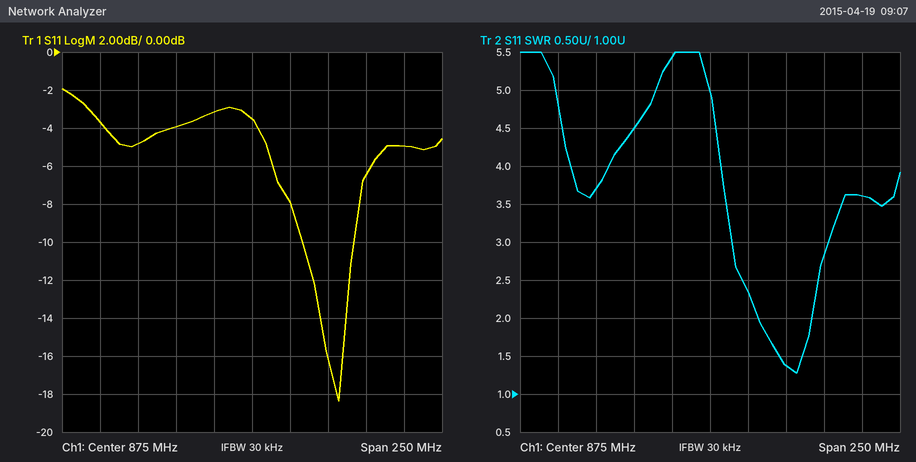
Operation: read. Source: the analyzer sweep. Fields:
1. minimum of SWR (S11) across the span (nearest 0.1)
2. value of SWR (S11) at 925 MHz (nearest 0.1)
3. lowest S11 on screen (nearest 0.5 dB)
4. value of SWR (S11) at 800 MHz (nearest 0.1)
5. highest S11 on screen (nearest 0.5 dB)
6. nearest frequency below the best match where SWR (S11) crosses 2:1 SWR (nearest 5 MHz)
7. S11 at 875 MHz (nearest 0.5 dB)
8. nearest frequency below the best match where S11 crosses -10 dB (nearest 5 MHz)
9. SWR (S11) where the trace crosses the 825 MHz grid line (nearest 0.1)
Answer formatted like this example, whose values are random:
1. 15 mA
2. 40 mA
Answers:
1. 1.3
2. 1.4
3. -18.5 dB
4. 3.7
5. -2.0 dB
6. 905 MHz
7. -3.5 dB
8. 910 MHz
9. 4.5
